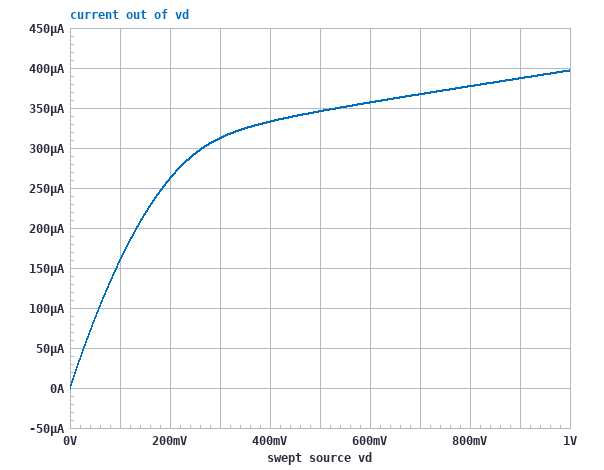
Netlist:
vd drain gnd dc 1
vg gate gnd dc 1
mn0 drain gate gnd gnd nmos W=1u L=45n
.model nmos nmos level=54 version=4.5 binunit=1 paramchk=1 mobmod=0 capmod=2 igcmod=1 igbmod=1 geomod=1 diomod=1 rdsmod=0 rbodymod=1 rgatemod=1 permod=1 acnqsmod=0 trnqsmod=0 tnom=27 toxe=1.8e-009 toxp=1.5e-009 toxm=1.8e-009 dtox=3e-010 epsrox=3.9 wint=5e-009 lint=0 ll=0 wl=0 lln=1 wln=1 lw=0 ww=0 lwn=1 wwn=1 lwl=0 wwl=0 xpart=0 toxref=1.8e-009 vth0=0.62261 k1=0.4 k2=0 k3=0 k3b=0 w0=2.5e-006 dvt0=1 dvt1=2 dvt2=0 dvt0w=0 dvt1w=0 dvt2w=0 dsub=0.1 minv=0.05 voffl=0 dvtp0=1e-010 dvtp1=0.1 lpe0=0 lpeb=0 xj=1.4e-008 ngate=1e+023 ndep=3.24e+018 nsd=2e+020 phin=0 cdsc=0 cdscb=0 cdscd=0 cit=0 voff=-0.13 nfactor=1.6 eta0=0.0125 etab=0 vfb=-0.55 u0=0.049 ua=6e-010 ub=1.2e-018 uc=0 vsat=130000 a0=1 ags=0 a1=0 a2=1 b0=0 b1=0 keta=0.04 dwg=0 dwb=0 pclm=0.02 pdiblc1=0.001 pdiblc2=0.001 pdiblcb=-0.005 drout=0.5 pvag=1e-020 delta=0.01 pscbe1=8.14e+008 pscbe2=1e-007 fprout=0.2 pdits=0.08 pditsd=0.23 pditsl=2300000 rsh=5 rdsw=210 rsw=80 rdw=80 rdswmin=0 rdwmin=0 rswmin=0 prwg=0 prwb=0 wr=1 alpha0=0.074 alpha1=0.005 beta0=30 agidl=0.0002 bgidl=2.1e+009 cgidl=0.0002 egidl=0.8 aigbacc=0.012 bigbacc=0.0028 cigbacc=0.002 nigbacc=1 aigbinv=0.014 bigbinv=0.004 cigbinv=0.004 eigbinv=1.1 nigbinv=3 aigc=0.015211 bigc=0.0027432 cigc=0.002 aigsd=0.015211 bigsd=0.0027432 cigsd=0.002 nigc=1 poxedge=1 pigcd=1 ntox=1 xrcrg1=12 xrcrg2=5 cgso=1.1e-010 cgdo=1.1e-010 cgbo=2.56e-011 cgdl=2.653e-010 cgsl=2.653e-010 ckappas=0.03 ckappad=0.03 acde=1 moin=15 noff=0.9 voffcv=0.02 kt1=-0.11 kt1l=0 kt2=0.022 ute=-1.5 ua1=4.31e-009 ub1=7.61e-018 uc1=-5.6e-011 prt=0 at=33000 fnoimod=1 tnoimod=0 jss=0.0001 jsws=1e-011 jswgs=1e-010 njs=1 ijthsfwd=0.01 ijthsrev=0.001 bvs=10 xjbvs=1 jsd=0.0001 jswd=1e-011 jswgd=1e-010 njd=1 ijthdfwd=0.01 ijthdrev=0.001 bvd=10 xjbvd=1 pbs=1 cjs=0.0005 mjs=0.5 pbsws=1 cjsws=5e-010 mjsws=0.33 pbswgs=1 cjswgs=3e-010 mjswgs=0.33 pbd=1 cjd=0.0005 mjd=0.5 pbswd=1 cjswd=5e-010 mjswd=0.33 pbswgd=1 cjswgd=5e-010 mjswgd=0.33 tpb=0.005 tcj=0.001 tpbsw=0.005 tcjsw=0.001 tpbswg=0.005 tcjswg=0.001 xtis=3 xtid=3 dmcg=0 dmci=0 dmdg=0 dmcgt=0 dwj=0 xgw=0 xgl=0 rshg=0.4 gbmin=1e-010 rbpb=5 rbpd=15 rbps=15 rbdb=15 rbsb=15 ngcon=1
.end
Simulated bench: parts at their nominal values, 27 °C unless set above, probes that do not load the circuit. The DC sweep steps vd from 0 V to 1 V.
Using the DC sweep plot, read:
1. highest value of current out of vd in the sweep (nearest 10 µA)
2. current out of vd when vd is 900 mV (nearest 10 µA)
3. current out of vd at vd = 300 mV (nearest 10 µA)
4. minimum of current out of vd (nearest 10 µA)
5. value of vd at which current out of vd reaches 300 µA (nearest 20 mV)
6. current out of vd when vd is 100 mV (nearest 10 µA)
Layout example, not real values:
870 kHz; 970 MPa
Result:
400 µA; 390 µA; 310 µA; 0 A; 260 mV; 160 µA
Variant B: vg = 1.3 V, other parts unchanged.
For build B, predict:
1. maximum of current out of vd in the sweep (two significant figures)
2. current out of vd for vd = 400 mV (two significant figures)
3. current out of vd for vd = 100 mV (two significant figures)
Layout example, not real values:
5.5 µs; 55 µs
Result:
730 µA; 610 µA; 220 µA
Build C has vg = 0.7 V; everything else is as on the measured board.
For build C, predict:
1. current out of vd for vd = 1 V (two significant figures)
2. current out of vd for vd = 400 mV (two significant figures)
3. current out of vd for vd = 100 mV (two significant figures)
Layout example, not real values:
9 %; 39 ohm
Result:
92 µA; 60 µA; 41 µA
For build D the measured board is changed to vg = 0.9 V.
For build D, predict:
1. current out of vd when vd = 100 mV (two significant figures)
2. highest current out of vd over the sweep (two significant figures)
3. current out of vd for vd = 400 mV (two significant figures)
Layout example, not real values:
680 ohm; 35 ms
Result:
130 µA; 290 µA; 230 µA
